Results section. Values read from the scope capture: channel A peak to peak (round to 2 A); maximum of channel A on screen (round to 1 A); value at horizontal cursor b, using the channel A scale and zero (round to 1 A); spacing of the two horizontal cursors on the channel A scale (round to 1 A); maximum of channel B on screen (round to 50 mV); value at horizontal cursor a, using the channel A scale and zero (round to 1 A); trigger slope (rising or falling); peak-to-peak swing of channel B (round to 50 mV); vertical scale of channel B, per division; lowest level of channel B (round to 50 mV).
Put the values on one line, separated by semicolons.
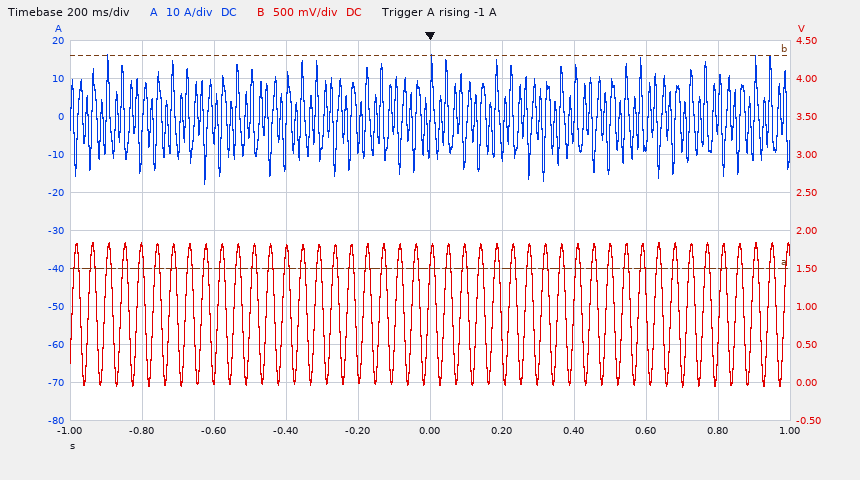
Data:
34 A; 16 A; 16 A; 56 A; 1.85 V; -40 A; rising; 1.90 V; 500 mV; -50 mV
